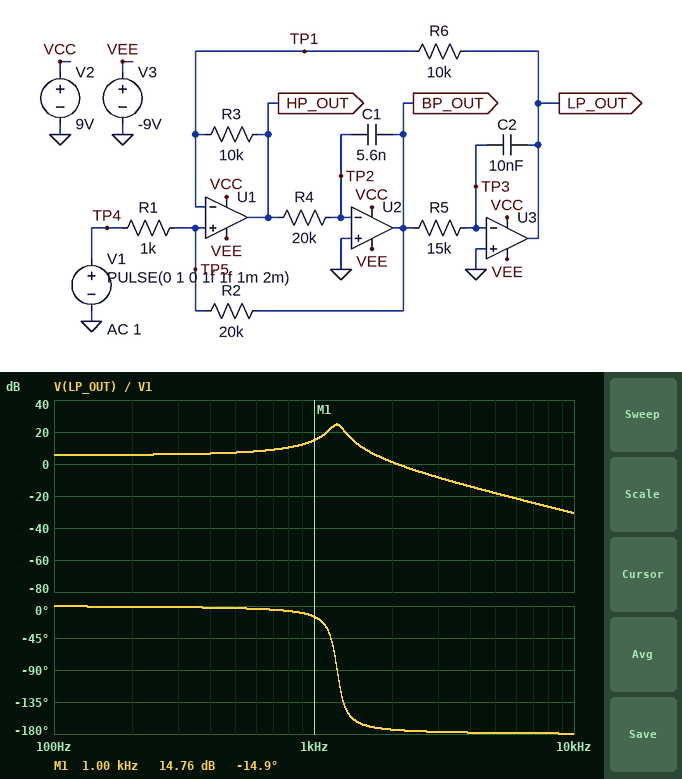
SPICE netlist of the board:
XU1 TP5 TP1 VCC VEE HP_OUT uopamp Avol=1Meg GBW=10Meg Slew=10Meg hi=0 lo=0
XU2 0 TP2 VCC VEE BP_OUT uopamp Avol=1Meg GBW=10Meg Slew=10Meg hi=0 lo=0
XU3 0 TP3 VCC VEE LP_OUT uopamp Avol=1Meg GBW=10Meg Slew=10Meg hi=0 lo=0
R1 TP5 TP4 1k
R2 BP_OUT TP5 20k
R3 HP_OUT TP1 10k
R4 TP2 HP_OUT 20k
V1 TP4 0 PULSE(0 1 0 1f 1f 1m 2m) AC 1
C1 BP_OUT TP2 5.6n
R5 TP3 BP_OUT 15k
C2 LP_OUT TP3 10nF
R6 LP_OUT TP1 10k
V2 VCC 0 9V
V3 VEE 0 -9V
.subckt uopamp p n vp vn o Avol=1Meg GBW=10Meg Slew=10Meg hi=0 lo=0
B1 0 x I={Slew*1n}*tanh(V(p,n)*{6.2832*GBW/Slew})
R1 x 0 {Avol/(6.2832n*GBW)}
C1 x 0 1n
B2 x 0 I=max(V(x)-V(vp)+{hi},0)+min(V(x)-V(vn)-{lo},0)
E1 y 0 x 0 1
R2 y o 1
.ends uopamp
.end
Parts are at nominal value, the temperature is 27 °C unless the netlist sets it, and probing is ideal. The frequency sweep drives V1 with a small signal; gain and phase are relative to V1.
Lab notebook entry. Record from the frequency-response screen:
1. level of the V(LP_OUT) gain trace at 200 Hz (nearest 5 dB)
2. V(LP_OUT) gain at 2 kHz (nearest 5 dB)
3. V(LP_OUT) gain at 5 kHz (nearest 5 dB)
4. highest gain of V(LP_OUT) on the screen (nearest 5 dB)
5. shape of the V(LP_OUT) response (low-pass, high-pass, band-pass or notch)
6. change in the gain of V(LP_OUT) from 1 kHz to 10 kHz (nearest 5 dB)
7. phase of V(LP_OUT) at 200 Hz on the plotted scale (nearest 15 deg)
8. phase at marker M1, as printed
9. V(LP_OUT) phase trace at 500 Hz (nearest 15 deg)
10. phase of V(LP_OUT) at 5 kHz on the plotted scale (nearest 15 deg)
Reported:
5 dB
0 dB
-20 dB
25 dB
low-pass
-45 dB
0 deg
-14.9 deg
0 deg
-180 deg
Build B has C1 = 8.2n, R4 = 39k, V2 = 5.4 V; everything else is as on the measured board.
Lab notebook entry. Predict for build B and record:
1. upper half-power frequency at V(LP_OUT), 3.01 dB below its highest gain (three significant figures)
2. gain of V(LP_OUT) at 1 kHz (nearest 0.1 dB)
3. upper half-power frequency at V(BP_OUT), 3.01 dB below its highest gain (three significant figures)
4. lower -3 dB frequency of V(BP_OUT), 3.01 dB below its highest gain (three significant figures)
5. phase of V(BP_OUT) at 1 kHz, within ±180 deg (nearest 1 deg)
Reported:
749 Hz
6.5 dB
751 Hz
703 Hz
96 deg
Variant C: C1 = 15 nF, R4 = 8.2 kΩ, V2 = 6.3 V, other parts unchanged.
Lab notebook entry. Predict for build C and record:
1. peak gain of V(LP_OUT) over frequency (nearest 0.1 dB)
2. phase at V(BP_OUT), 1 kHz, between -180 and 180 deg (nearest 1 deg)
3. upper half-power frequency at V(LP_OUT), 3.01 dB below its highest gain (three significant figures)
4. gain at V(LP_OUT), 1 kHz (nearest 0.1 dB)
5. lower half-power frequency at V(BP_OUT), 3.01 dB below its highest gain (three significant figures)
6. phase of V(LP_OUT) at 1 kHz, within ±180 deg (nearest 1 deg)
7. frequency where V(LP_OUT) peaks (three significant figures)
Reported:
25.2 dB
-108 deg
1.23 kHz
16.5 dB
1.11 kHz
-18 deg
1.17 kHz
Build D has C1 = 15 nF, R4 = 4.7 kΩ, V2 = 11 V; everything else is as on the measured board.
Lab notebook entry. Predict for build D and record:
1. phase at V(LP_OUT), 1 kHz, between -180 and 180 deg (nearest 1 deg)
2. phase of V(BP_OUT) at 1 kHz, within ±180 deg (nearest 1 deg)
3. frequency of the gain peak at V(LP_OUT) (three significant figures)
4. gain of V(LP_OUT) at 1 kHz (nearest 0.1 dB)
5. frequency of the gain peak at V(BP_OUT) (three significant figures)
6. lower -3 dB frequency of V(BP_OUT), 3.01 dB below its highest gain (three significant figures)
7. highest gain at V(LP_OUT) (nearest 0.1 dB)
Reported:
-9 deg
-99 deg
1.54 kHz
10.2 dB
1.55 kHz
1.44 kHz
22.8 dB
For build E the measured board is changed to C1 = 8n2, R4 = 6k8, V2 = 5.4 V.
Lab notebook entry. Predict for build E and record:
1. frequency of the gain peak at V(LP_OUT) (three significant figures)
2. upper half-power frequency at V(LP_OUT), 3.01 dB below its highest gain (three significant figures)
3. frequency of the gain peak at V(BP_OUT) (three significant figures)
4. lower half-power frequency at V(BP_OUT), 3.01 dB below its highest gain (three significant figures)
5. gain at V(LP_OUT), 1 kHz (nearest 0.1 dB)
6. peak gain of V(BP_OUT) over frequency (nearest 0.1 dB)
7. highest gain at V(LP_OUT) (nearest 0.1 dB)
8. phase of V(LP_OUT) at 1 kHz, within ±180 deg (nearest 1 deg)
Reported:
1.73 kHz
1.86 kHz
1.74 kHz
1.61 kHz
9.0 dB
26.1 dB
21.8 dB
-8 deg
